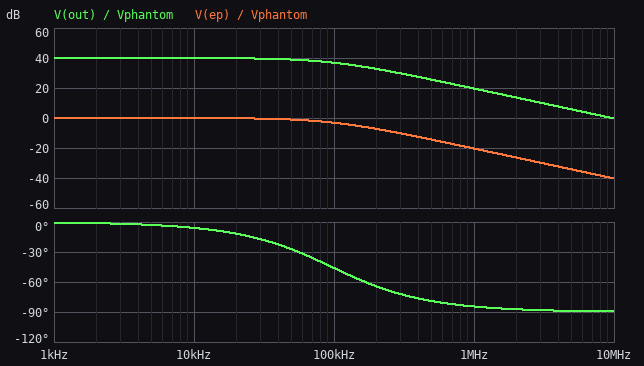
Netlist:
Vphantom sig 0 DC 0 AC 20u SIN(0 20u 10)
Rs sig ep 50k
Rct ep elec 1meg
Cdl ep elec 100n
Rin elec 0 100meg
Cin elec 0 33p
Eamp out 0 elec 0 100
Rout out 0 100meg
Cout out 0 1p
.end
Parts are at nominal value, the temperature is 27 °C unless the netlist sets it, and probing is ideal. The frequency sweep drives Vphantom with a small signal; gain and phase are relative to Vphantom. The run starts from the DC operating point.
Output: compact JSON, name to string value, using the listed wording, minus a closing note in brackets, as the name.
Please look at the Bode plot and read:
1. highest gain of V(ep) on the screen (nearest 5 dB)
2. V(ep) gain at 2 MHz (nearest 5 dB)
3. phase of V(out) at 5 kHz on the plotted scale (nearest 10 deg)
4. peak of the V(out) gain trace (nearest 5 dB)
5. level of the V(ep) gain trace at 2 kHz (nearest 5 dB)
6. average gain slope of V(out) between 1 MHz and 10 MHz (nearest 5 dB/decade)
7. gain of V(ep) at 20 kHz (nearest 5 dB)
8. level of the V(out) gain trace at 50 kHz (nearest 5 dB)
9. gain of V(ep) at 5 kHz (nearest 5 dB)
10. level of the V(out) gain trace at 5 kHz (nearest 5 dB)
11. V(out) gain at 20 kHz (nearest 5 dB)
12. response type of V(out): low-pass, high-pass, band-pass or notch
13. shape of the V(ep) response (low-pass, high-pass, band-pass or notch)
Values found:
{"highest gain of V(ep) on the screen": "0 dB", "V(ep) gain at 2 MHz": "-25 dB", "phase of V(out) at 5 kHz on the plotted scale": "0 deg", "peak of the V(out) gain trace": "40 dB", "level of the V(ep) gain trace at 2 kHz": "0 dB", "average gain slope of V(out) between 1 MHz and 10 MHz": "-20 dB/decade", "gain of V(ep) at 20 kHz": "0 dB", "level of the V(out) gain trace at 50 kHz": "40 dB", "gain of V(ep) at 5 kHz": "0 dB", "level of the V(out) gain trace at 5 kHz": "40 dB", "V(out) gain at 20 kHz": "40 dB", "response type of V(out): low-pass, high-pass, band-pass or notch": "low-pass", "shape of the V(ep) response": "low-pass"}
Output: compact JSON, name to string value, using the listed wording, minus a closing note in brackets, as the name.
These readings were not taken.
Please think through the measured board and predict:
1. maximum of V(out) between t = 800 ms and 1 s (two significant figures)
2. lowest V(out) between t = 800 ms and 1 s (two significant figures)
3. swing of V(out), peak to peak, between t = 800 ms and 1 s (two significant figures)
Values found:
{"maximum of V(out) between t = 800 ms and 1 s": "2.0 mV", "lowest V(out) between t = 800 ms and 1 s": "-2.0 mV", "swing of V(out), peak to peak, between t = 800 ms and 1 s": "4.0 mV"}
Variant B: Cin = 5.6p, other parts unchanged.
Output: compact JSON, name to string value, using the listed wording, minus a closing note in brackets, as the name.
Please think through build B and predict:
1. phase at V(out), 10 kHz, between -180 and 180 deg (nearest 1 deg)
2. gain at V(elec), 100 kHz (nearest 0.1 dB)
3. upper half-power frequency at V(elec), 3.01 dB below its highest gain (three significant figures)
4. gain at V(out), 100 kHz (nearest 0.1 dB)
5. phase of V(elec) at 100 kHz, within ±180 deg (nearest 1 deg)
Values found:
{"phase at V(out), 10 kHz, between -180 and 180 deg": "-1 deg", "gain at V(elec), 100 kHz": "-0.1 dB", "upper half-power frequency at V(elec), 3.01 dB below its highest gain": "569 kHz", "gain at V(out), 100 kHz": "39.9 dB", "phase of V(elec) at 100 kHz, within ±180 deg": "-10 deg"}
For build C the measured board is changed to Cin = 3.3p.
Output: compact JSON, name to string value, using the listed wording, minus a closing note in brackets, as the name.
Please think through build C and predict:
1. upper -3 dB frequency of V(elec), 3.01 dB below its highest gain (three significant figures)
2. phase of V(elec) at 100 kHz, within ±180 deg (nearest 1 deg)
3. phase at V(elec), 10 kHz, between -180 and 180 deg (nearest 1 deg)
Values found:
{"upper -3 dB frequency of V(elec), 3.01 dB below its highest gain": "965 kHz", "phase of V(elec) at 100 kHz, within ±180 deg": "-6 deg", "phase at V(elec), 10 kHz, between -180 and 180 deg": "-1 deg"}
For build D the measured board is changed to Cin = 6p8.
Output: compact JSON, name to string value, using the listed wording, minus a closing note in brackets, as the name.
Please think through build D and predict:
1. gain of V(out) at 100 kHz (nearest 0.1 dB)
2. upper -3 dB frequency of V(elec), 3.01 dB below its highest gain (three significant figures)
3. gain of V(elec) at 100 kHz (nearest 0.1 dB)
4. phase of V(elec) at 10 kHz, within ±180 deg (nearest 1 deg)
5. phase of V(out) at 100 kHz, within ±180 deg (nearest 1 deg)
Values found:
{"gain of V(out) at 100 kHz": "39.8 dB", "upper -3 dB frequency of V(elec), 3.01 dB below its highest gain": "468 kHz", "gain of V(elec) at 100 kHz": "-0.2 dB", "phase of V(elec) at 10 kHz, within ±180 deg": "-1 deg", "phase of V(out) at 100 kHz, within ±180 deg": "-12 deg"}
